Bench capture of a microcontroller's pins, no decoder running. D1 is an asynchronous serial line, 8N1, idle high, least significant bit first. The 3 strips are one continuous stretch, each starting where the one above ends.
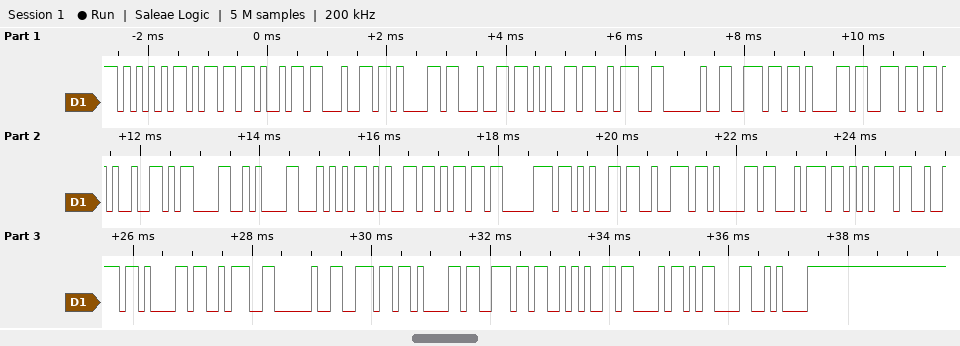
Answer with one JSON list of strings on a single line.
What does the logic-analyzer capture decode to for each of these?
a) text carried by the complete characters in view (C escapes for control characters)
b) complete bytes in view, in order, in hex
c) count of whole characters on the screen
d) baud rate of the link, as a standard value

["\"Umidade: nan%\\r\\nTemperatura: nan*C\\r\\n\"", "55 6D 69 64 61 64 65 3A 20 6E 61 6E 25 0D 0A 54 65 6D 70 65 72 61 74 75 72 61 3A 20 6E 61 6E 2A 43 0D 0A", "35", "9600 baud"]
